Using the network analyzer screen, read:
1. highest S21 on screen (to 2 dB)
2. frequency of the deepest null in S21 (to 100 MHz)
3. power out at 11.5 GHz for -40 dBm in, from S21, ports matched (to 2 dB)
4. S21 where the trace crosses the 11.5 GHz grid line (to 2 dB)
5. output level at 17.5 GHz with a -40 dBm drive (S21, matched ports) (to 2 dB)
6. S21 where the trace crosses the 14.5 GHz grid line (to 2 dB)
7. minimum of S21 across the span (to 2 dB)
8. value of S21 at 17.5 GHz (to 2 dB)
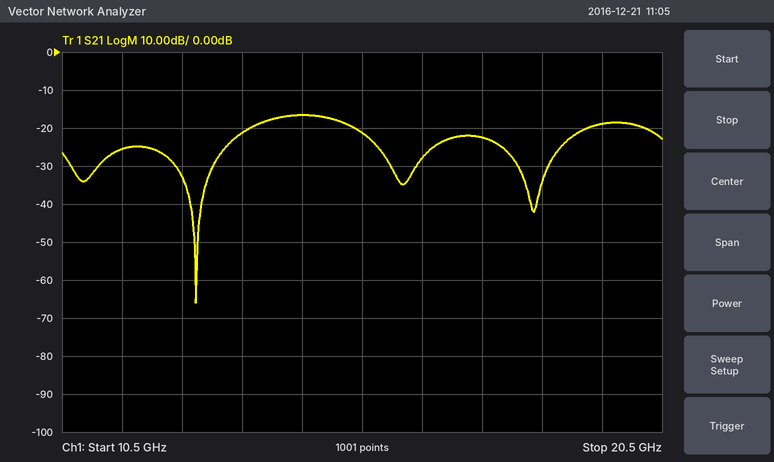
-16 dB
12.7 GHz
-66 dBm
-26 dB
-62 dBm
-16 dB
-66 dB
-22 dB
